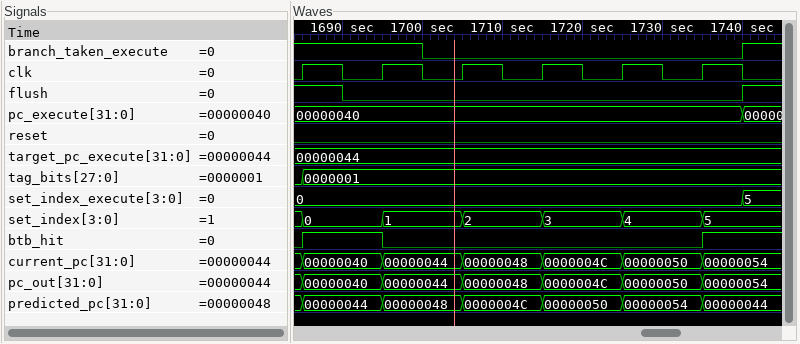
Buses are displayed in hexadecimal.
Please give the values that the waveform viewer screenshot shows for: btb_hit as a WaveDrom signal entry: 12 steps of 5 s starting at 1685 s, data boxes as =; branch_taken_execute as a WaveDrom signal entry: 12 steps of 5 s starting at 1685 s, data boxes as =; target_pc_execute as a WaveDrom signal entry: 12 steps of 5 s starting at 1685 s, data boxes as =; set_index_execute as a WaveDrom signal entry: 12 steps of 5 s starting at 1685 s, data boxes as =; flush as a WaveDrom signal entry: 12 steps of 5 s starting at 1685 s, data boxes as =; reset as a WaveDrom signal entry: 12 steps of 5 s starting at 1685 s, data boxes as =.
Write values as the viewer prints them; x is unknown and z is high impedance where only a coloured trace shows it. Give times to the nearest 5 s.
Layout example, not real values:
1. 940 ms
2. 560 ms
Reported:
1. {name: 'btb_hit', wave: '1.0.......1.'}
2. {name: 'branch_taken_execute', wave: '1..0.......1'}
3. {name: 'target_pc_execute', wave: '=...........', data: '00000044'}
4. {name: 'set_index_execute', wave: '=..........=', data: '0 5'}
5. {name: 'flush', wave: '10.........1'}
6. {name: 'reset', wave: '0...........'}
